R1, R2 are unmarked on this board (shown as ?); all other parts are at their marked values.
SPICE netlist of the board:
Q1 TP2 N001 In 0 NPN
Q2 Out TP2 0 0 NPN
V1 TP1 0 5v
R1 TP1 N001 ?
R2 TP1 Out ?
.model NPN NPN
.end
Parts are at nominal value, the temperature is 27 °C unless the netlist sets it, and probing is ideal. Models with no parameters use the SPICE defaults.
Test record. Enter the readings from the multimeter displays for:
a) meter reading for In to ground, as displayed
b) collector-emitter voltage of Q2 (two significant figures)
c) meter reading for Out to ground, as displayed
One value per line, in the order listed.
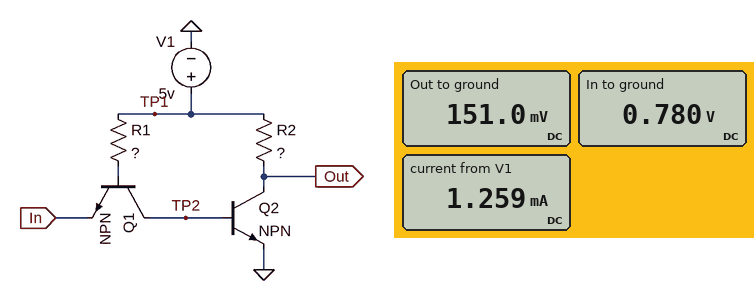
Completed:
0.780 V
150 mV
151.0 mV
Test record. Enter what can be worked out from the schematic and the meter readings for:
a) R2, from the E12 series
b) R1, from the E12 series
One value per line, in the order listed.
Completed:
3.9 kΩ
220 kΩ
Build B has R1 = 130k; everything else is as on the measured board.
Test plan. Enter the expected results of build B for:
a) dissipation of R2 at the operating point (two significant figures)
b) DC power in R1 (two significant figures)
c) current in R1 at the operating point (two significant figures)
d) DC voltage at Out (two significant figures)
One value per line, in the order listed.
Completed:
6.1 mW
96 µW
27 µA
120 mV
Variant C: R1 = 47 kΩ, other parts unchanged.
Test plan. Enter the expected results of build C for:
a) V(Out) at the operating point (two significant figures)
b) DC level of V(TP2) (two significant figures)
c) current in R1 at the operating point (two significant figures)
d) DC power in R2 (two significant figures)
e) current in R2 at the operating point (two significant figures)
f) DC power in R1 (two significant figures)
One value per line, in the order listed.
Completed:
81 mV
780 mV
75 µA
6.2 mW
1.3 mA
260 µW
